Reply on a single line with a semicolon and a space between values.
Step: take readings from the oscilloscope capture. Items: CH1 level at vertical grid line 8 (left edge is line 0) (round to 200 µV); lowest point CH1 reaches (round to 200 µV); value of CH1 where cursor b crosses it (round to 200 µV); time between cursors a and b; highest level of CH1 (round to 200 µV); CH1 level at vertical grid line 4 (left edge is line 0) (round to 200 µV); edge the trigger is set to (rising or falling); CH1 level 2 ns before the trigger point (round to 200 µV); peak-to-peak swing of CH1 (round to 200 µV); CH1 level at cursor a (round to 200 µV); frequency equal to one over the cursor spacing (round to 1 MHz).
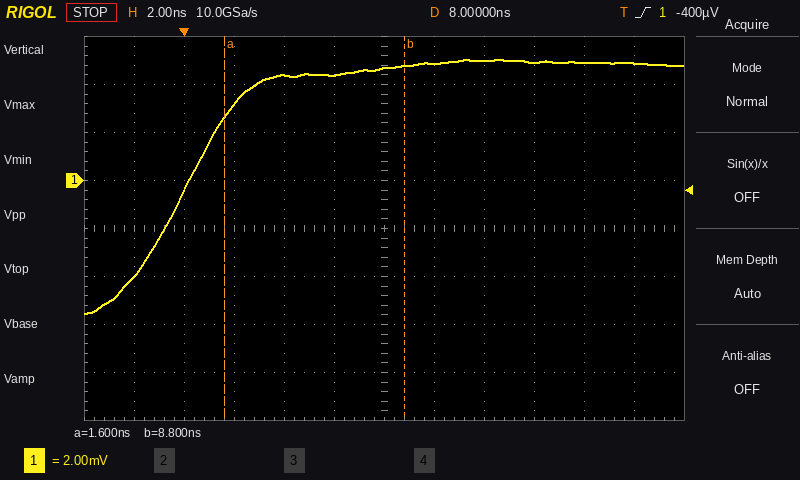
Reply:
5.0 mV; -5.6 mV; 4.8 mV; 7.2 ns; 5.0 mV; 4.4 mV; rising; -4.0 mV; 10.6 mV; 2.6 mV; 139 MHz
